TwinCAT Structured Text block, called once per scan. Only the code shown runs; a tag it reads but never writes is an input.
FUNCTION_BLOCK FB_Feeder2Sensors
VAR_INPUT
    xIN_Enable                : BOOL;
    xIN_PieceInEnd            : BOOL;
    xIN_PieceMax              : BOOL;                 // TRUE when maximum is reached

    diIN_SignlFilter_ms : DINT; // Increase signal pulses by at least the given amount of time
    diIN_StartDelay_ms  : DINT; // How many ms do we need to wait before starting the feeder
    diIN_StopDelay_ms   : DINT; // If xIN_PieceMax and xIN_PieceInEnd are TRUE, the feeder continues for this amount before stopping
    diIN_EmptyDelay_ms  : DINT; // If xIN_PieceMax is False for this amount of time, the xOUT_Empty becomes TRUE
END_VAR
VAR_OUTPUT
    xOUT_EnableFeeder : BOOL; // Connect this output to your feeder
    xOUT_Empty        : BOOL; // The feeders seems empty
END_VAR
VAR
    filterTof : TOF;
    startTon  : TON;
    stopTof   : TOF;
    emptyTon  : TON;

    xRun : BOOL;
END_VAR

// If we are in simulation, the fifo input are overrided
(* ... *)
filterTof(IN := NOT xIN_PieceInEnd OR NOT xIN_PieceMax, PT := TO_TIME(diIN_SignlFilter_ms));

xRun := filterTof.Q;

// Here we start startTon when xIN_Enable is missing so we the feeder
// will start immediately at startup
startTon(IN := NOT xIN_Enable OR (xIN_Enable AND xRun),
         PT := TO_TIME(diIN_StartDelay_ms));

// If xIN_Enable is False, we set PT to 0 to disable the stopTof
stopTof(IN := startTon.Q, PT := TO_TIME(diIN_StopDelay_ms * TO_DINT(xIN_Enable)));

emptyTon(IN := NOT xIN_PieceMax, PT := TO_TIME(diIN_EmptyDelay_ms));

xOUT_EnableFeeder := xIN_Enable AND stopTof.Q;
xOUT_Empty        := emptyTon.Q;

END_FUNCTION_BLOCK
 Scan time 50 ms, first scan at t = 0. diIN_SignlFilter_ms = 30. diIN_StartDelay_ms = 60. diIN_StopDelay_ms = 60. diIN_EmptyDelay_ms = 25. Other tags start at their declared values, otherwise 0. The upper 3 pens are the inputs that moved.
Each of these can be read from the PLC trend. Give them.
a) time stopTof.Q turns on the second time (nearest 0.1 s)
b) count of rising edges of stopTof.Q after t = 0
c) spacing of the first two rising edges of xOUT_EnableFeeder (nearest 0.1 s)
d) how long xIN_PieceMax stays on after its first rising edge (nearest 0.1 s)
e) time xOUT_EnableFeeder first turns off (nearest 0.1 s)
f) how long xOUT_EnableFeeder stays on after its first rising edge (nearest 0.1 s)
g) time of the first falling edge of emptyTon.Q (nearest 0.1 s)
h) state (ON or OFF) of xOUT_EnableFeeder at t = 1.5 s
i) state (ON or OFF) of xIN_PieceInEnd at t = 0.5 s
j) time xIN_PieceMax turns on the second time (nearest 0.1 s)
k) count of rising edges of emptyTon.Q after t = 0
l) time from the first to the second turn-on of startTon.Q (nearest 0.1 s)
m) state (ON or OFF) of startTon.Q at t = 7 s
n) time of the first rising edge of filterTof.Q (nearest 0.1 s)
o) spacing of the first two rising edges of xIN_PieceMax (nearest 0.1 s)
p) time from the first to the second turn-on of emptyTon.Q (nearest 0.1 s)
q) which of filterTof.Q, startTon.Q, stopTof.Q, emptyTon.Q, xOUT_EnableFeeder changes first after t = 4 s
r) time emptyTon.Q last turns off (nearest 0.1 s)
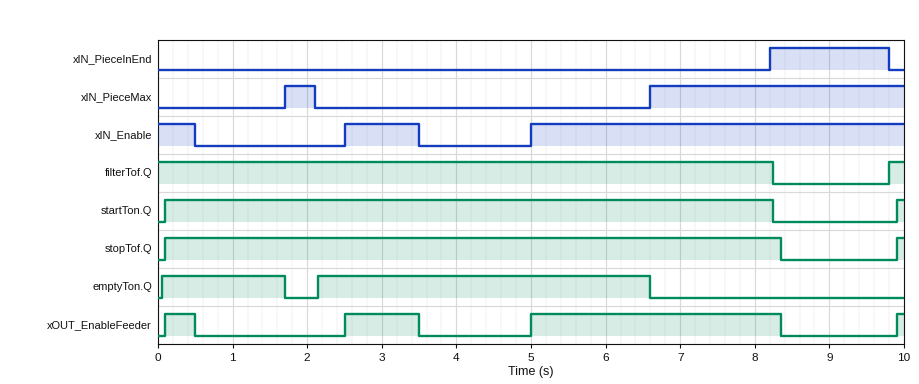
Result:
9.9 s
2
2.4 s
0.4 s
0.5 s
0.4 s
1.7 s
OFF
OFF
6.6 s
2
9.8 s
ON
9.8 s
4.9 s
2.1 s
xOUT_EnableFeeder
6.6 s
